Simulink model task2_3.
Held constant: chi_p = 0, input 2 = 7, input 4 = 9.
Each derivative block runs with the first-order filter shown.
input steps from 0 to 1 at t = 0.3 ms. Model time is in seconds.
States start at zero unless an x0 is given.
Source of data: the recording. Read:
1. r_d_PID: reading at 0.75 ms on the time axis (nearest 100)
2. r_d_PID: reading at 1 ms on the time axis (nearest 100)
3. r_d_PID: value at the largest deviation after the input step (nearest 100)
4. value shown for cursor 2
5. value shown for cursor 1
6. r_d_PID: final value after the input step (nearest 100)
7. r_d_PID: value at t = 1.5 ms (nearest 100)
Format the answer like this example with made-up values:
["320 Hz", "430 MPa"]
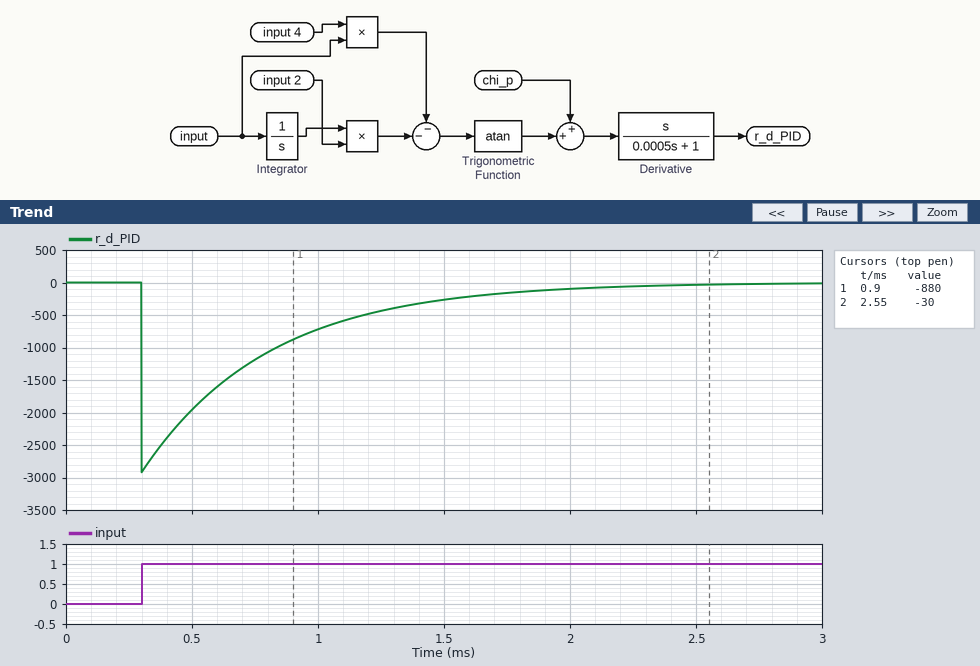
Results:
["-1200", "-700", "-2900", "-30", "-880", "0", "-300"]
